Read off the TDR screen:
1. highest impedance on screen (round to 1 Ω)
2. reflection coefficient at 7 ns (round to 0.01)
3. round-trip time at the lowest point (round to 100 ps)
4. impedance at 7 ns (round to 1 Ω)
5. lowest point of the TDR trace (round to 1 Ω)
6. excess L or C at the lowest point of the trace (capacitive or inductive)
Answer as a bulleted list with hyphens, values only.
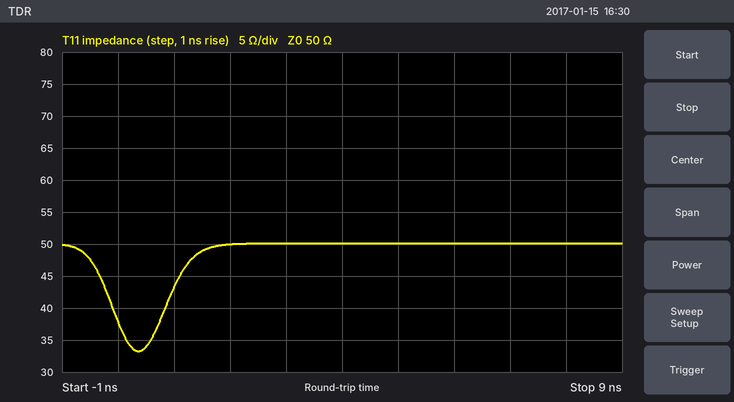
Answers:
- 50 Ω
- 0.00
- 400 ps
- 50 Ω
- 33 Ω
- capacitive
